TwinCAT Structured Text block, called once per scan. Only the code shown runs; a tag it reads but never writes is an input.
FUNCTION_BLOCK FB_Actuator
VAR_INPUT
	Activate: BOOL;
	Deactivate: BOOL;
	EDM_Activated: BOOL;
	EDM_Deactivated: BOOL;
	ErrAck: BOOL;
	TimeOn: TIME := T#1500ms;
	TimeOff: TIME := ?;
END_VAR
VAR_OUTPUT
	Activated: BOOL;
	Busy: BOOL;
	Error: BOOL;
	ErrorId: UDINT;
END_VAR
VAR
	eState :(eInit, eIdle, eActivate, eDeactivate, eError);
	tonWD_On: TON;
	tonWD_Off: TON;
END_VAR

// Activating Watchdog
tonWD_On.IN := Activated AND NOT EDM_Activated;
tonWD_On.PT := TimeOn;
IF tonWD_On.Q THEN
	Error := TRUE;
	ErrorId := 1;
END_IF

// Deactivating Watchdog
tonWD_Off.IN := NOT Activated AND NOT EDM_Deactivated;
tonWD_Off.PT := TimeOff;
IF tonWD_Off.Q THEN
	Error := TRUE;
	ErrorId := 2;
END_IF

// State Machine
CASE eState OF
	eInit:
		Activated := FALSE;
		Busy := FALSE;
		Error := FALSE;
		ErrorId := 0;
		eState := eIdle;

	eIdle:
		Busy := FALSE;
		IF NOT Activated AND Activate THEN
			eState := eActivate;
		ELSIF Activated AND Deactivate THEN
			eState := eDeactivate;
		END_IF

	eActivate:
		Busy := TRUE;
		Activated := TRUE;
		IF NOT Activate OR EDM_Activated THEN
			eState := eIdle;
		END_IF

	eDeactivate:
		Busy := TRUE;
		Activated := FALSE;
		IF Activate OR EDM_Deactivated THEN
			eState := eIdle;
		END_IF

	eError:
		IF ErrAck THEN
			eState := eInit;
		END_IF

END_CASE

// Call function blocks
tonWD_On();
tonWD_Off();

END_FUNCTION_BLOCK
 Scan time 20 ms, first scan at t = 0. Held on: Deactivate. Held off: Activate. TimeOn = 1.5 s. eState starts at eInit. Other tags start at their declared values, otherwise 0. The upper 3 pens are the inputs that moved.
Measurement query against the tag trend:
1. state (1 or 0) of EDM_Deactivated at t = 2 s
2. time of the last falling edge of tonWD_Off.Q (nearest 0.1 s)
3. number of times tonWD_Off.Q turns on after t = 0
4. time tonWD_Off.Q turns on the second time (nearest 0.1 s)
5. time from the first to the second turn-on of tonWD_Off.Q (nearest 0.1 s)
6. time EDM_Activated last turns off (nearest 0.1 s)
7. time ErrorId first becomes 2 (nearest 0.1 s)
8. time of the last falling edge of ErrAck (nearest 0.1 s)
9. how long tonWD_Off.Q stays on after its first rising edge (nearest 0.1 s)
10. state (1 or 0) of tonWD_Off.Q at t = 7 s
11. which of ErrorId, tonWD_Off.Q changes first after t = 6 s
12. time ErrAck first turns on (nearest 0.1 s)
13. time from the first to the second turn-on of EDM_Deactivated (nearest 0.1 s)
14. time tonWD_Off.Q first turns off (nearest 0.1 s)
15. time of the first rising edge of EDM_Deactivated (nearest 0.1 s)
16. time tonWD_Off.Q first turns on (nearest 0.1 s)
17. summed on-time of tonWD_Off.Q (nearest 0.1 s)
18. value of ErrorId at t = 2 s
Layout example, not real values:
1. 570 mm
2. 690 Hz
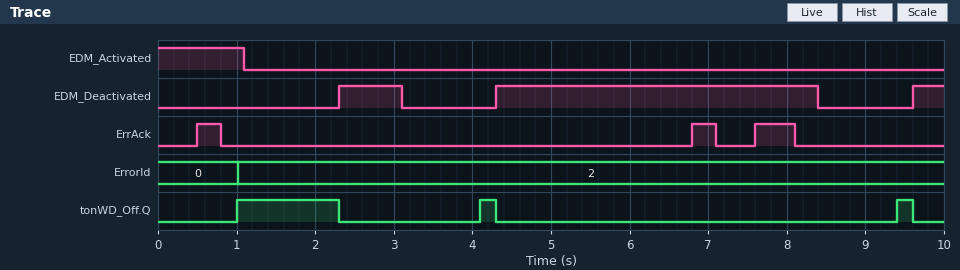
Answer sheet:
1. 0
2. 9.6 s
3. 3
4. 4.1 s
5. 3.1 s
6. 1.1 s
7. 1.0 s
8. 8.1 s
9. 1.3 s
10. 0
11. tonWD_Off.Q
12. 0.5 s
13. 2.0 s
14. 2.3 s
15. 2.3 s
16. 1.0 s
17. 1.7 s
18. 2
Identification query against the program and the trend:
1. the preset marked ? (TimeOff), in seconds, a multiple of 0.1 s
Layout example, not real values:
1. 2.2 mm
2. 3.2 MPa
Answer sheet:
1. 1.0 s
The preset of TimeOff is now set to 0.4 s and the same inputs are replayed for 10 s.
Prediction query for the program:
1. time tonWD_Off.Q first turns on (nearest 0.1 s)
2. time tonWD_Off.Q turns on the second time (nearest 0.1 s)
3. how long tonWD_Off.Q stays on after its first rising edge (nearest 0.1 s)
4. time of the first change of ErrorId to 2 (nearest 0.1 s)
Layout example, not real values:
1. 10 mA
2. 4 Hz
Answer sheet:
1. 0.4 s
2. 3.5 s
3. 1.9 s
4. 0.4 s
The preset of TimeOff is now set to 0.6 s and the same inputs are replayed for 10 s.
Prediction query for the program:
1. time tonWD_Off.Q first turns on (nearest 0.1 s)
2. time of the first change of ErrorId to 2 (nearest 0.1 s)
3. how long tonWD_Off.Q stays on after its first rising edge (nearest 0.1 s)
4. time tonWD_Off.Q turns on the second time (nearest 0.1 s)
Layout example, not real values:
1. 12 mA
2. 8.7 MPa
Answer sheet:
1. 0.6 s
2. 0.6 s
3. 1.7 s
4. 3.7 s
